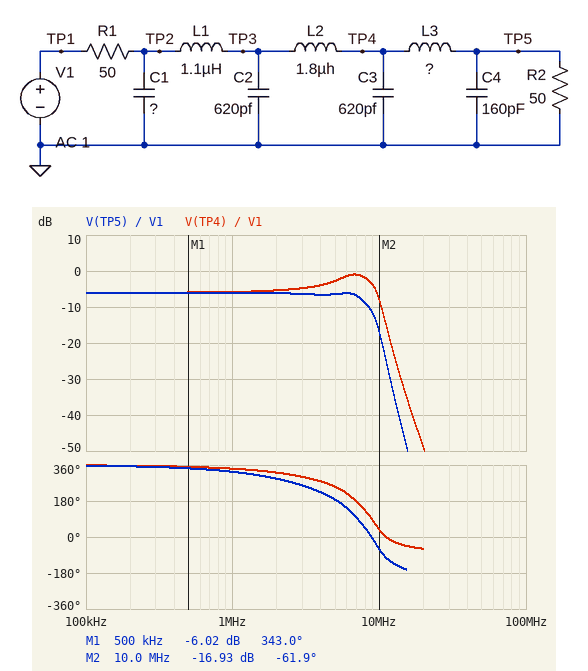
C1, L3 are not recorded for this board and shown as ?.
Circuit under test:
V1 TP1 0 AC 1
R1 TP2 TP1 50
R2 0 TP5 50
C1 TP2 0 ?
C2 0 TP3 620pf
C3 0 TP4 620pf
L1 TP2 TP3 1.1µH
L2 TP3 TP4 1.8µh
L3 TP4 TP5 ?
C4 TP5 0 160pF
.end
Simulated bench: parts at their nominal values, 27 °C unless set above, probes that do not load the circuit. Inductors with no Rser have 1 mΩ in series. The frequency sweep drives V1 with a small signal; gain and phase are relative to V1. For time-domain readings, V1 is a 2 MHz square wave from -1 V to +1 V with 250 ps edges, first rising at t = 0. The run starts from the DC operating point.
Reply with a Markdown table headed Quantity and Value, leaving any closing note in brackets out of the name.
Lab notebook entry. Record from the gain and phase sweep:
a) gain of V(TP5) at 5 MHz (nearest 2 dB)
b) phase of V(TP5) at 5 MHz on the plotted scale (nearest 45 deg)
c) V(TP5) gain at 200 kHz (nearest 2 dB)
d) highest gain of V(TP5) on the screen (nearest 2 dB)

| Quantity | Value |
|---|---|
| gain of V(TP5) at 5 MHz | -6 dB |
| phase of V(TP5) at 5 MHz on the plotted scale | 180 deg |
| V(TP5) gain at 200 kHz | -6 dB |
| highest gain of V(TP5) on the screen | -6 dB |
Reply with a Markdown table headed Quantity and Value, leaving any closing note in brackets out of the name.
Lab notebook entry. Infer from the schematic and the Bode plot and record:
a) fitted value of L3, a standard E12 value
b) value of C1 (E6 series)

| Quantity | Value |
|---|---|
| fitted value of L3, a standard E12 value | 2.2 µH |
| value of C1 | 330 pF |
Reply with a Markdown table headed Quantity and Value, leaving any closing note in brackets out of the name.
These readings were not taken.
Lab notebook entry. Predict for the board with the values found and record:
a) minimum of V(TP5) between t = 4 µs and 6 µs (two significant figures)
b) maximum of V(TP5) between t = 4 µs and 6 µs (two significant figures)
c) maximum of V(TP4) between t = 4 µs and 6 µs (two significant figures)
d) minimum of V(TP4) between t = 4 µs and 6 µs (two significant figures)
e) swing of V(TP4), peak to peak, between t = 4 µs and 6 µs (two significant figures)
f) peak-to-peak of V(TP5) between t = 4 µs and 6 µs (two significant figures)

| Quantity | Value |
|---|---|
| minimum of V(TP5) between t = 4 µs and 6 µs | -630 mV |
| maximum of V(TP5) between t = 4 µs and 6 µs | 630 mV |
| maximum of V(TP4) between t = 4 µs and 6 µs | 930 mV |
| minimum of V(TP4) between t = 4 µs and 6 µs | -930 mV |
| swing of V(TP4), peak to peak, between t = 4 µs and 6 µs | 1.9 V |
| peak-to-peak of V(TP5) between t = 4 µs and 6 µs | 1.3 V |
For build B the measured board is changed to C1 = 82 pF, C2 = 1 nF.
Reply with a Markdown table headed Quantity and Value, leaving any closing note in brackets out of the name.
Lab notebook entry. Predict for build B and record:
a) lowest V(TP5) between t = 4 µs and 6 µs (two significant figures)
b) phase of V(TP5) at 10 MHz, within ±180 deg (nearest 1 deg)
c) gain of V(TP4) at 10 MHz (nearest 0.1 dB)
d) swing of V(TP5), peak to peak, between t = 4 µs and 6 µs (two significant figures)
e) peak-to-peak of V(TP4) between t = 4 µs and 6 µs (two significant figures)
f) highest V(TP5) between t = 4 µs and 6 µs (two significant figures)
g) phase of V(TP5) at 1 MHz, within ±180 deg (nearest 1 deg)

| Quantity | Value |
|---|---|
| lowest V(TP5) between t = 4 µs and 6 µs | -580 mV |
| phase of V(TP5) at 10 MHz, within ±180 deg | -54 deg |
| gain of V(TP4) at 10 MHz | -18.1 dB |
| swing of V(TP5), peak to peak, between t = 4 µs and 6 µs | 1.2 V |
| peak-to-peak of V(TP4) between t = 4 µs and 6 µs | 1.6 V |
| highest V(TP5) between t = 4 µs and 6 µs | 580 mV |
| phase of V(TP5) at 1 MHz, within ±180 deg | -35 deg |
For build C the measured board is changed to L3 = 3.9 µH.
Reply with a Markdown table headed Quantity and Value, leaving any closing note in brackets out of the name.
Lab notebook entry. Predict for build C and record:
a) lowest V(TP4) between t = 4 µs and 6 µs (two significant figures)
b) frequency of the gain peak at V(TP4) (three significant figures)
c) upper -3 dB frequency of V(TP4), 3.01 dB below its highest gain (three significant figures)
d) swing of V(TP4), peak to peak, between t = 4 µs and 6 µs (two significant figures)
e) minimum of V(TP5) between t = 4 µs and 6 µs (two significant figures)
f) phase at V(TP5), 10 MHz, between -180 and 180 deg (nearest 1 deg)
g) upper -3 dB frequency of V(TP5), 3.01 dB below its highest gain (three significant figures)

| Quantity | Value |
|---|---|
| lowest V(TP4) between t = 4 µs and 6 µs | -1.2 V |
| frequency of the gain peak at V(TP4) | 6.01 MHz |
| upper -3 dB frequency of V(TP4), 3.01 dB below its highest gain | 7.83 MHz |
| swing of V(TP4), peak to peak, between t = 4 µs and 6 µs | 2.4 V |
| minimum of V(TP5) between t = 4 µs and 6 µs | -540 mV |
| phase at V(TP5), 10 MHz, between -180 and 180 deg | -77 deg |
| upper -3 dB frequency of V(TP5), 3.01 dB below its highest gain | 6.33 MHz |
